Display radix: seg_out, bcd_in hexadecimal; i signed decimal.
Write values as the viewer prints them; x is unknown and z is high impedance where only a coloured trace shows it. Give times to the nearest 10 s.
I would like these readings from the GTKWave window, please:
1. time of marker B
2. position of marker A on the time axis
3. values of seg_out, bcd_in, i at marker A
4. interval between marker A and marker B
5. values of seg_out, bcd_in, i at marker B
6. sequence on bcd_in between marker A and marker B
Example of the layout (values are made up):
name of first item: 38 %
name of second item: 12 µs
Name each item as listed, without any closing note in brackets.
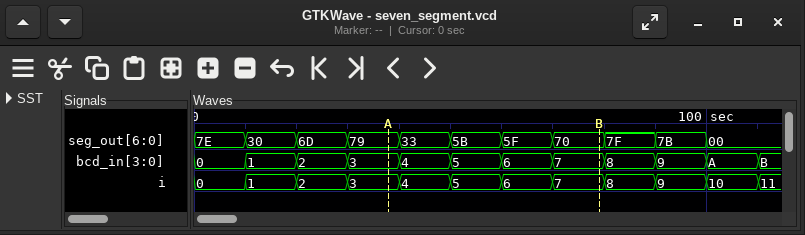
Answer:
time of marker B: 80 s
position of marker A on the time axis: 40 s
values of seg_out, bcd_in, i at marker A: seg_out=79, bcd_in=3, i=3
interval between marker A and marker B: 40 s
values of seg_out, bcd_in, i at marker B: seg_out=70, bcd_in=7, i=7
sequence on bcd_in between marker A and marker B: 3, 4, 5, 6, 7
